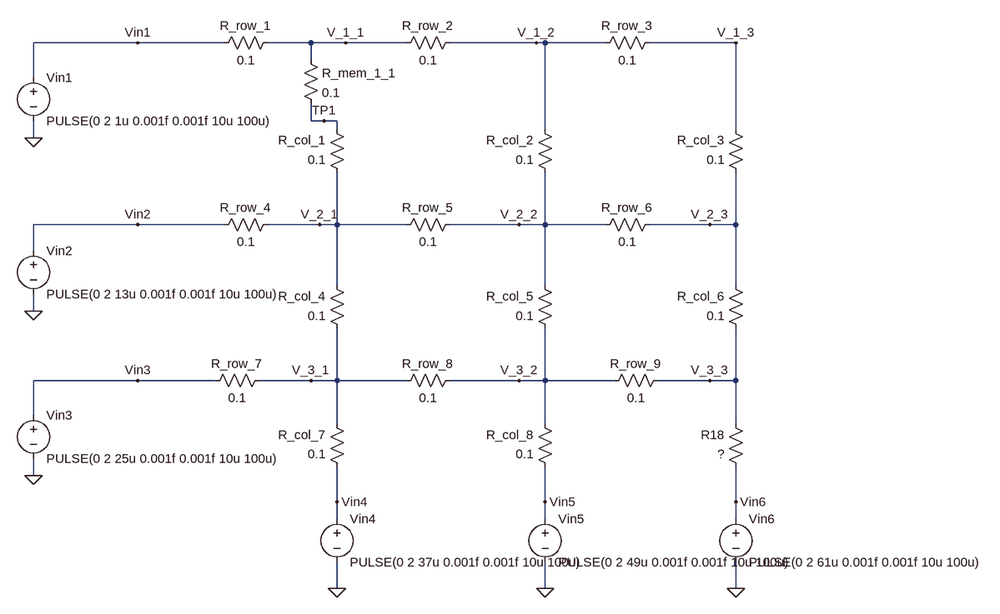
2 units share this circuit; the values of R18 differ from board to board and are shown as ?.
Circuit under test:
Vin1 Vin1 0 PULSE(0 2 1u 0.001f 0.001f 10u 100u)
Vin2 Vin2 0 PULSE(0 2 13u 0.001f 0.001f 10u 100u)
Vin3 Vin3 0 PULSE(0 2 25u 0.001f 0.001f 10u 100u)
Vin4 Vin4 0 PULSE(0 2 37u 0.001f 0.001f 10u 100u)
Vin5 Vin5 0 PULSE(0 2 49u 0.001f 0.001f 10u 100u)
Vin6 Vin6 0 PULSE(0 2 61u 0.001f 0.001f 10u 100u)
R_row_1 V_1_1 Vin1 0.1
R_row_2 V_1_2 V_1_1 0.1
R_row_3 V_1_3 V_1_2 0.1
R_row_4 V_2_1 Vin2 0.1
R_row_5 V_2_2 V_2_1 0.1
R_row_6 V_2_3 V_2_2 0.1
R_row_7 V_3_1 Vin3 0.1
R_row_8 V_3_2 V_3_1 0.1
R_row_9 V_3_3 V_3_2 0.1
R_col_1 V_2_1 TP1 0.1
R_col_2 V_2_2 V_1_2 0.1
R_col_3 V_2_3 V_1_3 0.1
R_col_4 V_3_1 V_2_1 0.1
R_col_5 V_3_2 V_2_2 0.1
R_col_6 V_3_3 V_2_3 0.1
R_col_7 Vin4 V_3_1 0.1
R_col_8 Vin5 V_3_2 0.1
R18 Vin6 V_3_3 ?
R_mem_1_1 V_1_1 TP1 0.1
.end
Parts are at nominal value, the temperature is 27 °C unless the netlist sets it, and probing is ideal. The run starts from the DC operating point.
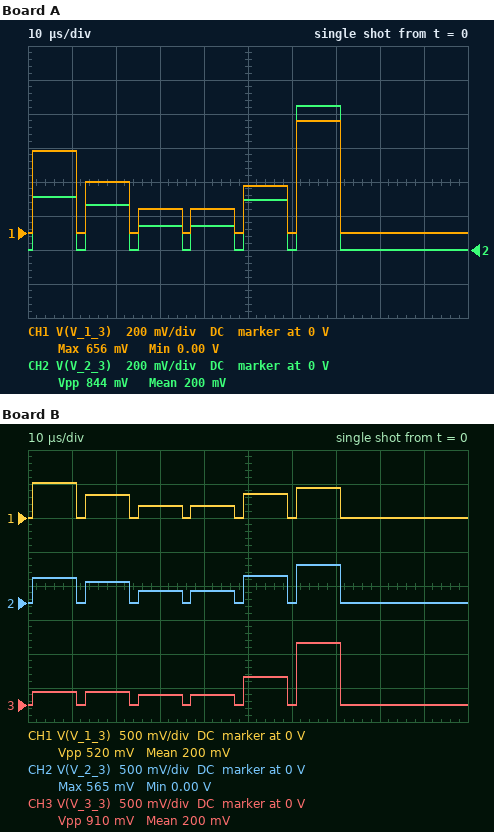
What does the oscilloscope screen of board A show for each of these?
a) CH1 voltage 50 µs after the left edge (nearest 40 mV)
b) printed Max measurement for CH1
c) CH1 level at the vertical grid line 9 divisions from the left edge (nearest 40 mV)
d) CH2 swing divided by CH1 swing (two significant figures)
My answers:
280 mV
656 mV
0 V
1.3
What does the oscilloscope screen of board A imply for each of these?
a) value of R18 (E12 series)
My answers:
0.047 Ω
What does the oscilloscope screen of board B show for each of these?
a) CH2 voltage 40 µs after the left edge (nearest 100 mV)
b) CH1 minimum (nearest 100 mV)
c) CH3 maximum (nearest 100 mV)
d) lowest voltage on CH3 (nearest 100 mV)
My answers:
200 mV
0 V
900 mV
0 V
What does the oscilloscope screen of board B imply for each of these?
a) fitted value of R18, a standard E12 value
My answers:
0.12 Ω
